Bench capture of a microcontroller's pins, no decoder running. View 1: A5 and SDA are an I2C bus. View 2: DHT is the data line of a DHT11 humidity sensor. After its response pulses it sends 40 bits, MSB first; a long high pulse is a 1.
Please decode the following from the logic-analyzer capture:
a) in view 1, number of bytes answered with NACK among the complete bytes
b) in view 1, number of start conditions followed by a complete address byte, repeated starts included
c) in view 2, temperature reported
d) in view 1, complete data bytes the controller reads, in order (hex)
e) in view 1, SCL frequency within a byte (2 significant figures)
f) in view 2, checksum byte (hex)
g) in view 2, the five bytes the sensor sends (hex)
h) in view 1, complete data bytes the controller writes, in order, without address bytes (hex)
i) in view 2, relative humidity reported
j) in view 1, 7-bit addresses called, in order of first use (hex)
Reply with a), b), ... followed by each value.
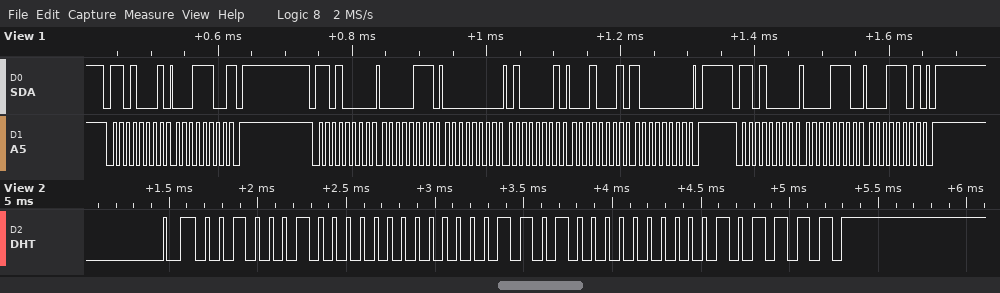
a) 1
b) 3
c) 13.0 °C
d) 1C
e) 100 kHz
f) 0x2F
g) 22 00 0D 00 2F
h) 07 00 41 11 80 0E 1D
i) 34 %
j) 0x68
